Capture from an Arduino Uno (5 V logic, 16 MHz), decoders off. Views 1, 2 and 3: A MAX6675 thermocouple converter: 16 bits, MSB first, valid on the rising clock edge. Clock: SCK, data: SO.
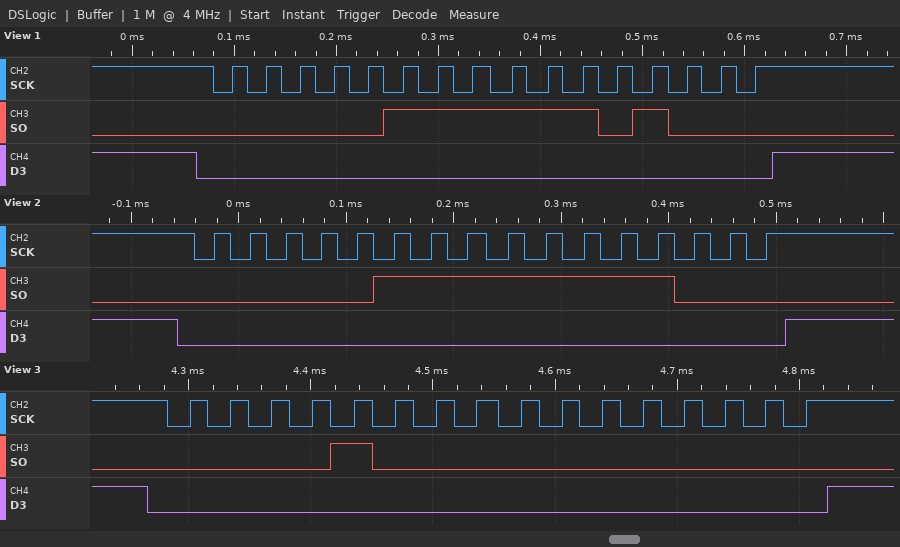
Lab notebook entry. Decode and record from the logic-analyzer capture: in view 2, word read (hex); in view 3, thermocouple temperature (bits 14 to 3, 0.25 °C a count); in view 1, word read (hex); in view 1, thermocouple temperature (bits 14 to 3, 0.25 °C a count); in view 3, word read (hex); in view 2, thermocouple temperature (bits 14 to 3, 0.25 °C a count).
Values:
0x07F8
64.00 °C
0x07E8
63.25 °C
0x0800
63.75 °C
